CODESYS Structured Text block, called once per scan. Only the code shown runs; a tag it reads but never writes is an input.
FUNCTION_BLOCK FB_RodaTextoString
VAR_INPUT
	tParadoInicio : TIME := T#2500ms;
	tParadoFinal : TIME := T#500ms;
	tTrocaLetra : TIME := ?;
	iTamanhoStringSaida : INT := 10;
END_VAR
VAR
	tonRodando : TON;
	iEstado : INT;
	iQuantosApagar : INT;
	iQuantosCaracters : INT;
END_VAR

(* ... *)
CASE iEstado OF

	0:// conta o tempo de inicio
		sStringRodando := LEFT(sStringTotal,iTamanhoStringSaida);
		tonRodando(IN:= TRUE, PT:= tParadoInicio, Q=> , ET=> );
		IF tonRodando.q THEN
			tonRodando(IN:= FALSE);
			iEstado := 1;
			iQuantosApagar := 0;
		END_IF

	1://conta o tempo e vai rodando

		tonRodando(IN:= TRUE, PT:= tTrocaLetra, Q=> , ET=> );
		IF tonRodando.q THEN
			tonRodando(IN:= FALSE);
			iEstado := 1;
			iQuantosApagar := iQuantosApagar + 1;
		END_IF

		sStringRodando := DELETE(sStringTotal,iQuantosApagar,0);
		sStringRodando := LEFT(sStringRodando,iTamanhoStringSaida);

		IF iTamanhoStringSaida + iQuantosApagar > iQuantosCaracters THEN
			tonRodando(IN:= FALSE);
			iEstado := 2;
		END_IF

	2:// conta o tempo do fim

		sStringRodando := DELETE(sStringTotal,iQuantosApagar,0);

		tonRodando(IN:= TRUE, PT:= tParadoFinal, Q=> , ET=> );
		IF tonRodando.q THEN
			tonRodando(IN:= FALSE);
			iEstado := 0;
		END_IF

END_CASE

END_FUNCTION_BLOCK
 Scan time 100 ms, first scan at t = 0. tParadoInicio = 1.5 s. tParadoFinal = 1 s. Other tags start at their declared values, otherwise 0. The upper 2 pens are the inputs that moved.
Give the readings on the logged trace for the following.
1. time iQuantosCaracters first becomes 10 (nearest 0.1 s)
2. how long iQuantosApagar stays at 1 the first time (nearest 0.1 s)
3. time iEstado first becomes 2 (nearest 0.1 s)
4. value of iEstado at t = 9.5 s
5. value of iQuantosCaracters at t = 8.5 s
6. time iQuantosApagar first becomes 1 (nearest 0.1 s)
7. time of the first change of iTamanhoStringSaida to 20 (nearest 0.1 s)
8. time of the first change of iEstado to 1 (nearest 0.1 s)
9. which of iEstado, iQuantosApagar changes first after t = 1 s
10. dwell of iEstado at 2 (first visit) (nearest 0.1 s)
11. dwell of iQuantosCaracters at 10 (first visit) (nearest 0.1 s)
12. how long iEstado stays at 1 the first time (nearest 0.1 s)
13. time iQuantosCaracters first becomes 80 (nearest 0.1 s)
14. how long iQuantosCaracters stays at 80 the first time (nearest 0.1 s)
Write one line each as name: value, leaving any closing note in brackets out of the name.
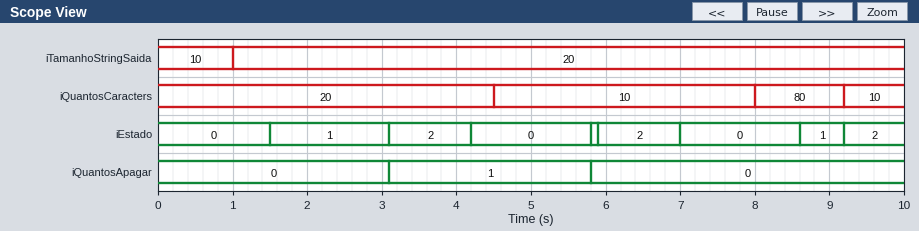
time iQuantosCaracters first becomes 10: 4.5 s
how long iQuantosApagar stays at 1 the first time: 2.7 s
time iEstado first becomes 2: 3.1 s
value of iEstado at t = 9.5 s: 2
value of iQuantosCaracters at t = 8.5 s: 80
time iQuantosApagar first becomes 1: 3.1 s
time of the first change of iTamanhoStringSaida to 20: 1.0 s
time of the first change of iEstado to 1: 1.5 s
which of iEstado, iQuantosApagar changes first after t = 1 s: iEstado
dwell of iEstado at 2 (first visit): 1.1 s
dwell of iQuantosCaracters at 10 (first visit): 3.5 s
how long iEstado stays at 1 the first time: 1.6 s
time iQuantosCaracters first becomes 80: 8.0 s
how long iQuantosCaracters stays at 80 the first time: 1.2 s
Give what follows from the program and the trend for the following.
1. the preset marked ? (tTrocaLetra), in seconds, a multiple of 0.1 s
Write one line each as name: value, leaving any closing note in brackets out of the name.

the preset marked ? (tTrocaLetra), in seconds, a multiple of 0.1 s: 1.5 s
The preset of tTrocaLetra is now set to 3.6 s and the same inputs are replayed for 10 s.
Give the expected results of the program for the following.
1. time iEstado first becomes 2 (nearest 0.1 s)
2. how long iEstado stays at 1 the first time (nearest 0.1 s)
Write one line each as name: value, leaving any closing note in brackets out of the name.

time iEstado first becomes 2: 4.5 s
how long iEstado stays at 1 the first time: 3.0 s
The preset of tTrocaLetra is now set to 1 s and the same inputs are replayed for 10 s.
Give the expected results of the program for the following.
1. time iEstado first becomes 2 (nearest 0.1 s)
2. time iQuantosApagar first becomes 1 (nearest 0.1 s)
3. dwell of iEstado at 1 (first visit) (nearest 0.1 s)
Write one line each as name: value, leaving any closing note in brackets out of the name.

time iEstado first becomes 2: 2.6 s
time iQuantosApagar first becomes 1: 2.6 s
dwell of iEstado at 1 (first visit): 1.1 s
